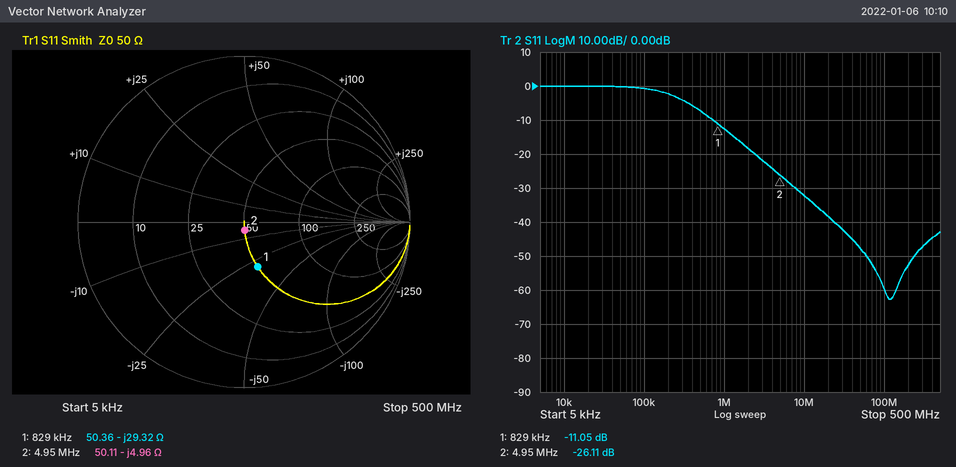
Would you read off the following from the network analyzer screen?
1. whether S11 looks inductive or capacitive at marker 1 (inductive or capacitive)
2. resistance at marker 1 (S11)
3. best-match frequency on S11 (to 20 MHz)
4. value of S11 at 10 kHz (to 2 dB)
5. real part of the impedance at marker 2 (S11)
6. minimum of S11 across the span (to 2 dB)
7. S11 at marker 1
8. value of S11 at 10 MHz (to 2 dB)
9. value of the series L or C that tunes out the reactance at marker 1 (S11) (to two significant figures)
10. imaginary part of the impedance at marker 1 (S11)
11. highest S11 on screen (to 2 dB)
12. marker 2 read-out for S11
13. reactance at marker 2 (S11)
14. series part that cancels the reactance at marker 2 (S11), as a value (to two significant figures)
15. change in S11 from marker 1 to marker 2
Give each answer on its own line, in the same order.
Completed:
capacitive
50.36 Ω
120 MHz
0 dB
50.11 Ω
-62 dB
-11.05 dB
-32 dB
5.6 µH
-29.32 Ω
0 dB
-26.11 dB
-4.96 Ω
160 nH
-15.06 dB
